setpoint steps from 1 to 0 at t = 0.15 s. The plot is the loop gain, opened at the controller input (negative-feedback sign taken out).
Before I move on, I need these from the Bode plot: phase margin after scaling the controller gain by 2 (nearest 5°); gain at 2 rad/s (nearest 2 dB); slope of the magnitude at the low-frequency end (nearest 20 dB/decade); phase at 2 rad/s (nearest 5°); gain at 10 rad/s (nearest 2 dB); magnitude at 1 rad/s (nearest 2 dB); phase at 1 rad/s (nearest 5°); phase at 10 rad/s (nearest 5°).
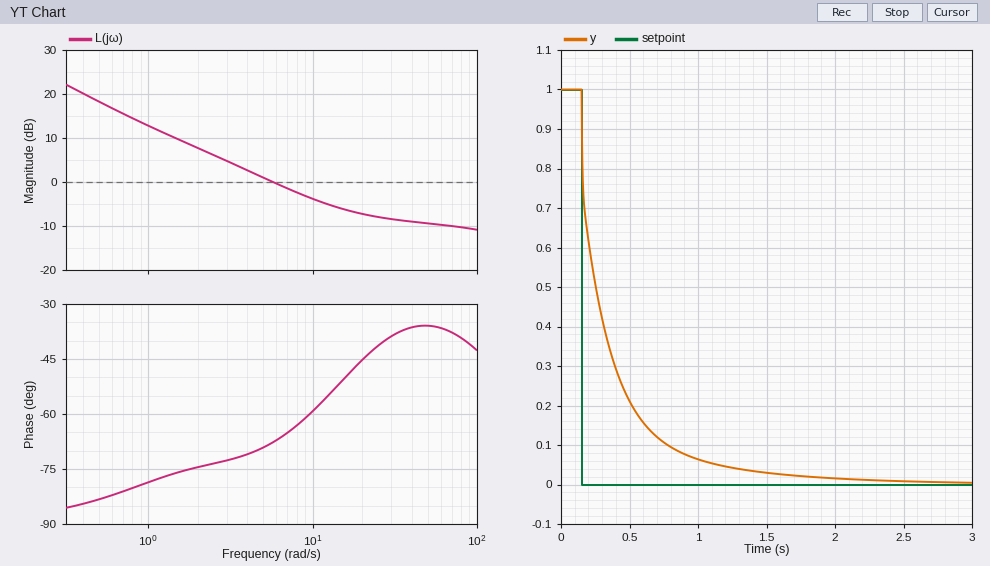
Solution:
130°
8 dB
-20 dB/decade
-75°
-4 dB
12 dB
-80°
-60°
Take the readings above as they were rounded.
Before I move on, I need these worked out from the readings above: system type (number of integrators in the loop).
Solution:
1
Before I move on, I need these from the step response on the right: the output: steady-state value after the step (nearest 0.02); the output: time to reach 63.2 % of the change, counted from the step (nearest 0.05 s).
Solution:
0.00
0.20 s
